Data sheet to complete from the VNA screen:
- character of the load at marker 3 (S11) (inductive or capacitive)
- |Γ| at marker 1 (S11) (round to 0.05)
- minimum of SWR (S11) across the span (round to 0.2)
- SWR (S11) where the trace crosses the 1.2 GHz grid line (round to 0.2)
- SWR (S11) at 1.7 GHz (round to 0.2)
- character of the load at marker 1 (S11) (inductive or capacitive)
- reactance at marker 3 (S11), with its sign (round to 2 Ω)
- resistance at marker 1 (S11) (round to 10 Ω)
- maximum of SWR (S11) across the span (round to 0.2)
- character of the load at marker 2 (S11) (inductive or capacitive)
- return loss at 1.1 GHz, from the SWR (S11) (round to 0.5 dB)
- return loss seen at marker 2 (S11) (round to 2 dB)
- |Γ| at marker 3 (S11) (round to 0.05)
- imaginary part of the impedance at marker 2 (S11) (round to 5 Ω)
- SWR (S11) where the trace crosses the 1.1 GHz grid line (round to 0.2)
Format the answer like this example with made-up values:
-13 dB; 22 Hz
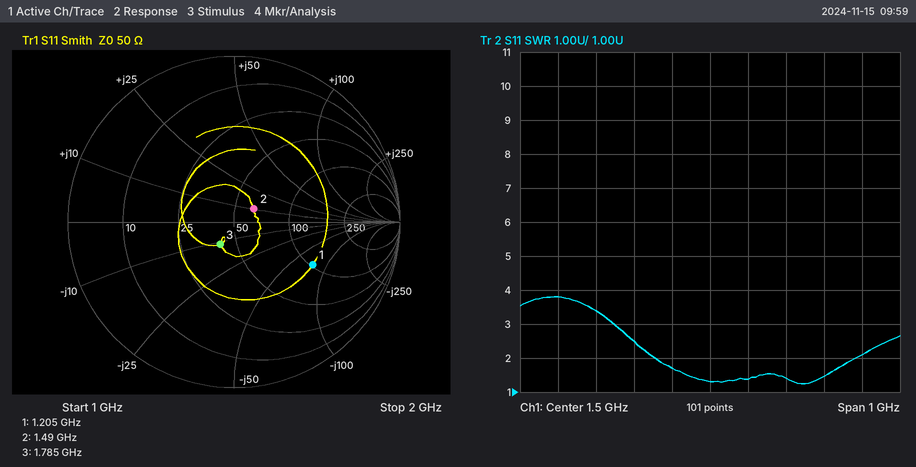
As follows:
capacitive; 0.55; 1.2; 3.4; 1.4; capacitive; -12 Ω; 100 Ω; 3.8; inductive; 4.5 dB; 16 dB; 0.15; +10 Ω; 3.8
